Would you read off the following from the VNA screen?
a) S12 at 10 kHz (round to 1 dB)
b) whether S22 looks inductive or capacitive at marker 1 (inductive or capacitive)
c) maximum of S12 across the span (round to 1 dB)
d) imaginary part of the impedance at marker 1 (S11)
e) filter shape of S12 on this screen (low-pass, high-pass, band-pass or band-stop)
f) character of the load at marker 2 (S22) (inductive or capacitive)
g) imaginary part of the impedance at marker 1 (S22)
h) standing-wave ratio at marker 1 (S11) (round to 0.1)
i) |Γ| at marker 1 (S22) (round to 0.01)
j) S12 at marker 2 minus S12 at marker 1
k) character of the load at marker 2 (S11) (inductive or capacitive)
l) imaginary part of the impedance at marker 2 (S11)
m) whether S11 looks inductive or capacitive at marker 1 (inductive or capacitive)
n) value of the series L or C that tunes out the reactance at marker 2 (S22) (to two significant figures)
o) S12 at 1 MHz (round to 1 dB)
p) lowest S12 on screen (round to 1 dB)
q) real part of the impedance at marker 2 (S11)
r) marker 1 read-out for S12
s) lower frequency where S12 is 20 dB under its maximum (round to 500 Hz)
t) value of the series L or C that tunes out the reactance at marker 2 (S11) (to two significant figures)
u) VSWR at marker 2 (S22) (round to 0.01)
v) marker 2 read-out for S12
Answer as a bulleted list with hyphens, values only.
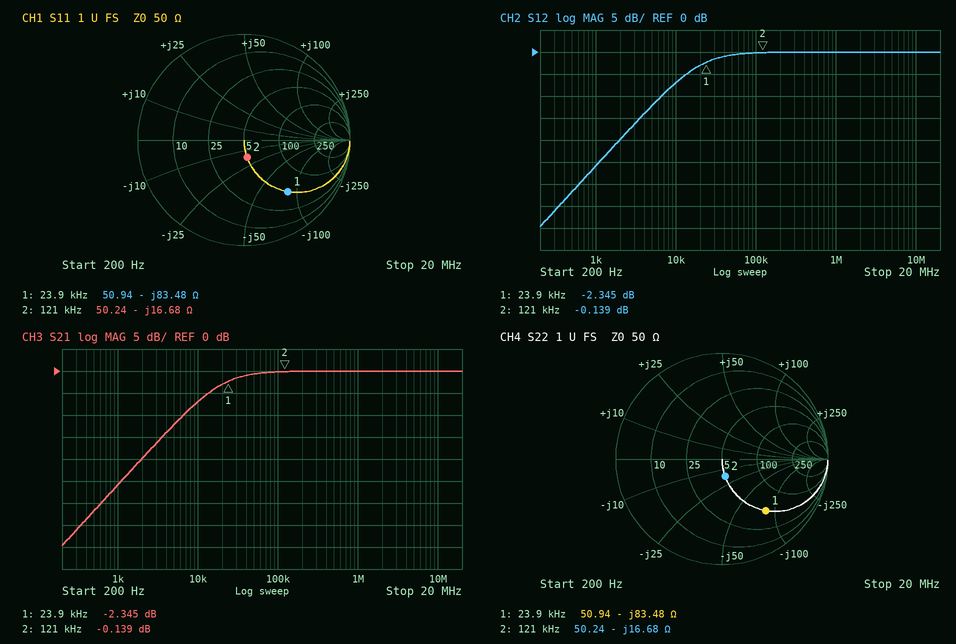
- -7 dB
- capacitive
- 0 dB
- -83.48 Ω
- high-pass
- capacitive
- -83.48 Ω
- 4.5
- 0.64
- 2.206 dB
- capacitive
- -16.68 Ω
- capacitive
- 22 µH
- 0 dB
- -40 dB
- 50.24 Ω
- -2.345 dB
- 2.0 kHz
- 22 µH
- 1.39
- -0.139 dB
